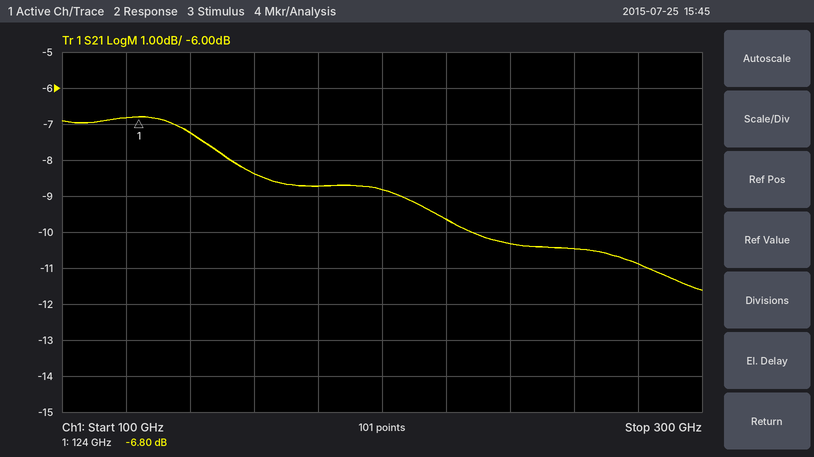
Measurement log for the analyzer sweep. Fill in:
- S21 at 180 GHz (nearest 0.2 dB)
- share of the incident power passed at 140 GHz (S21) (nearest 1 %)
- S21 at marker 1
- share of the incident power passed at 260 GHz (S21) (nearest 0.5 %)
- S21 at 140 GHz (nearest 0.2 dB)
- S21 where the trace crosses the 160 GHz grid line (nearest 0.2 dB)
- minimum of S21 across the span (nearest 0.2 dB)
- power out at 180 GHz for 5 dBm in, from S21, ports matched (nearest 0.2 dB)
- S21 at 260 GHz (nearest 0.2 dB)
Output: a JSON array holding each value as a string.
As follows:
["-8.8 dB", "19 %", "-6.80 dB", "9.0 %", "-7.2 dB", "-8.4 dB", "-11.6 dB", "-3.8 dBm", "-10.4 dB"]
